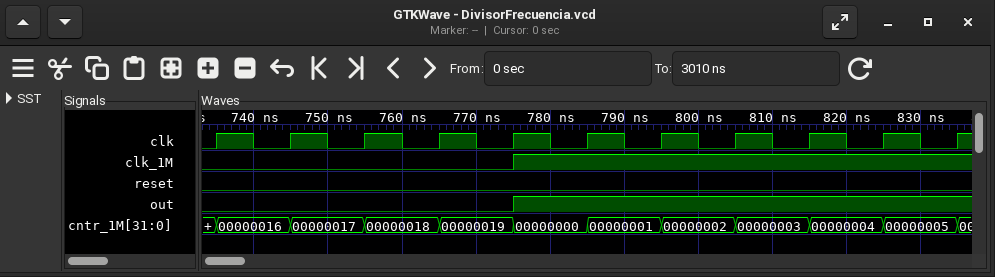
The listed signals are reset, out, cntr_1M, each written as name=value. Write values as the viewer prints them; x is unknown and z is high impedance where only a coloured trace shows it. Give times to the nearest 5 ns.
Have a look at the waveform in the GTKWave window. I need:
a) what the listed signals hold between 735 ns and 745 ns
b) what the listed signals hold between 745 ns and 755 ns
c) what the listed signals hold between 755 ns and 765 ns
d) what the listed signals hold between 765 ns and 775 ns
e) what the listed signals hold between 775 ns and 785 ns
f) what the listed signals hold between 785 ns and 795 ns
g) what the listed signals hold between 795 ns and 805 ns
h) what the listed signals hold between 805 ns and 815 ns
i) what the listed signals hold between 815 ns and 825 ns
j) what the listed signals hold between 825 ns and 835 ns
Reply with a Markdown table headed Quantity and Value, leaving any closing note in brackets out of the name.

| Quantity | Value |
|---|---|
| what the listed signals hold between 735 ns and 745 ns | reset=0, out=0, cntr_1M=00000016 |
| what the listed signals hold between 745 ns and 755 ns | reset=0, out=0, cntr_1M=00000017 |
| what the listed signals hold between 755 ns and 765 ns | reset=0, out=0, cntr_1M=00000018 |
| what the listed signals hold between 765 ns and 775 ns | reset=0, out=0, cntr_1M=00000019 |
| what the listed signals hold between 775 ns and 785 ns | reset=0, out=1, cntr_1M=00000000 |
| what the listed signals hold between 785 ns and 795 ns | reset=0, out=1, cntr_1M=00000001 |
| what the listed signals hold between 795 ns and 805 ns | reset=0, out=1, cntr_1M=00000002 |
| what the listed signals hold between 805 ns and 815 ns | reset=0, out=1, cntr_1M=00000003 |
| what the listed signals hold between 815 ns and 825 ns | reset=0, out=1, cntr_1M=00000004 |
| what the listed signals hold between 825 ns and 835 ns | reset=0, out=1, cntr_1M=00000005 |
